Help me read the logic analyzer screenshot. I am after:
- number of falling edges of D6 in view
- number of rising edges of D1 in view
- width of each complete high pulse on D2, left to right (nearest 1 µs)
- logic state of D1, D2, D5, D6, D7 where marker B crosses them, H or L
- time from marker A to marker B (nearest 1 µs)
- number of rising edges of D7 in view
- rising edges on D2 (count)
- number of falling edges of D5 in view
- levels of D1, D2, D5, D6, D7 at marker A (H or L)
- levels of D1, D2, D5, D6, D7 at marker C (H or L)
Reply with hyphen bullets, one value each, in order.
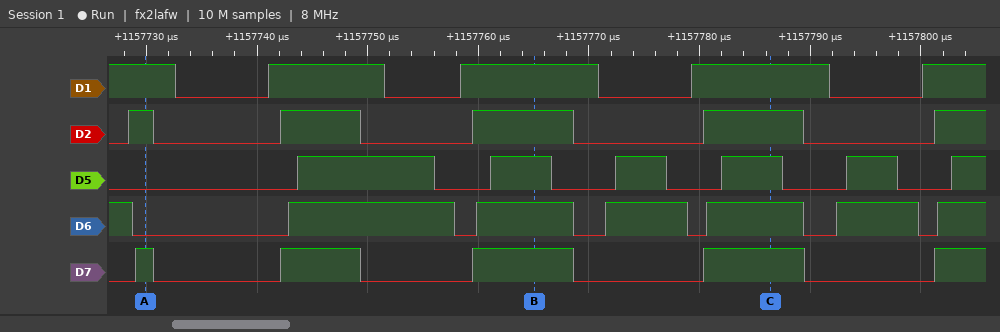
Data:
- 6
- 4
- 2 µs, 7 µs, 9 µs, 9 µs
- D1=H, D2=H, D5=H, D6=H, D7=H
- 35 µs
- 5
- 5
- 5
- D1=H, D2=H, D5=L, D6=L, D7=H
- D1=H, D2=H, D5=H, D6=H, D7=H
